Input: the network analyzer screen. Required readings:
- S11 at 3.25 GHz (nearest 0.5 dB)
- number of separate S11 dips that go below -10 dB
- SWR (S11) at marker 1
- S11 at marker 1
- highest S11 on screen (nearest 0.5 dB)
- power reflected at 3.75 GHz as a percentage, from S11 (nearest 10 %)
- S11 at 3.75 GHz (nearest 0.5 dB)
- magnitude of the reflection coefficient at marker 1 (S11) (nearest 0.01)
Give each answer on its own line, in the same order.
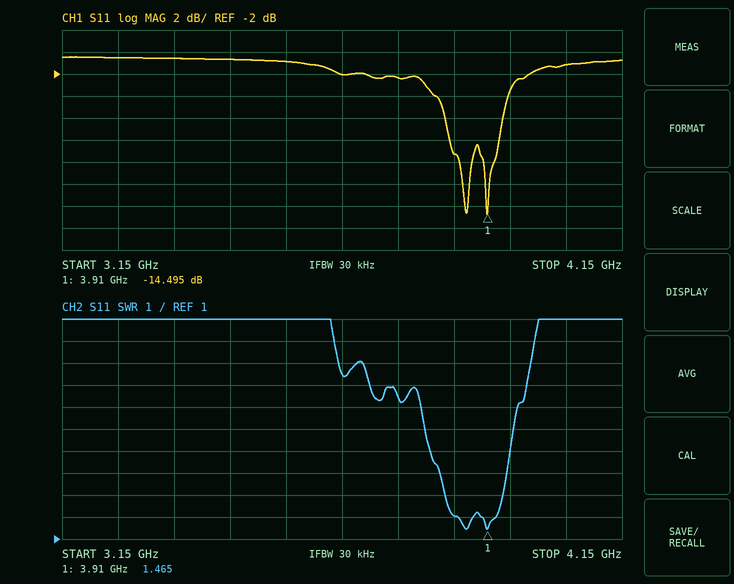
-0.5 dB
2
1.465
-14.495 dB
-0.5 dB
60 %
-2.5 dB
0.19
